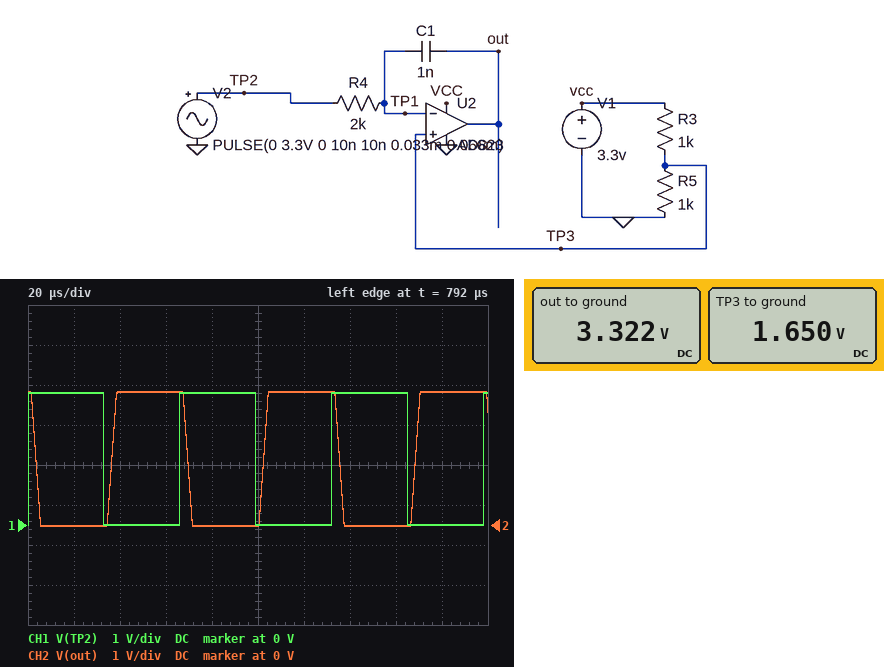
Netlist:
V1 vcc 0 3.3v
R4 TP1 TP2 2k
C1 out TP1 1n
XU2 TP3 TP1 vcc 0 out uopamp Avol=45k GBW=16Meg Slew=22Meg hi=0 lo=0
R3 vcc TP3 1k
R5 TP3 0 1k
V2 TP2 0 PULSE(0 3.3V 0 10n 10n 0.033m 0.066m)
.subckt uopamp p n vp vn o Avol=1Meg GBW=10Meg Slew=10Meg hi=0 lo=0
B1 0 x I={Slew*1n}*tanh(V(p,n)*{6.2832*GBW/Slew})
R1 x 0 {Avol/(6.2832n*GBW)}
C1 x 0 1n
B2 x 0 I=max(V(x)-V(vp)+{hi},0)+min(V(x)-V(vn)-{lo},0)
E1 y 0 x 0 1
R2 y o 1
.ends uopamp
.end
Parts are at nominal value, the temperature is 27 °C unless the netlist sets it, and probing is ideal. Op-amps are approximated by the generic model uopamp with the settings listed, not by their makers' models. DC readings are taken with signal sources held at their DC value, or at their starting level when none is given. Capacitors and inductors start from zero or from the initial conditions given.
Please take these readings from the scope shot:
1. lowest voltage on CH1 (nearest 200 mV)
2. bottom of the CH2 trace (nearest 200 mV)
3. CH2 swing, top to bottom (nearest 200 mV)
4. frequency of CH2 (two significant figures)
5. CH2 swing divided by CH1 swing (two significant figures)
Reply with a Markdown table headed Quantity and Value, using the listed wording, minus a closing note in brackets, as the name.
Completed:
| Quantity | Value |
|---|---|
| lowest voltage on CH1 | 0 V |
| bottom of the CH2 trace | 0 V |
| CH2 swing, top to bottom | 3.4 V |
| frequency of CH2 | 15 kHz |
| CH2 swing divided by CH1 swing | 1.0 |
